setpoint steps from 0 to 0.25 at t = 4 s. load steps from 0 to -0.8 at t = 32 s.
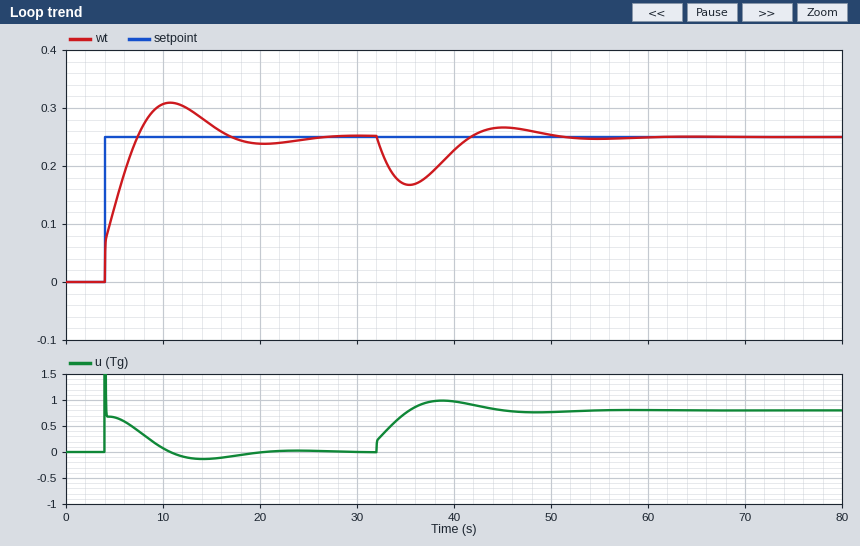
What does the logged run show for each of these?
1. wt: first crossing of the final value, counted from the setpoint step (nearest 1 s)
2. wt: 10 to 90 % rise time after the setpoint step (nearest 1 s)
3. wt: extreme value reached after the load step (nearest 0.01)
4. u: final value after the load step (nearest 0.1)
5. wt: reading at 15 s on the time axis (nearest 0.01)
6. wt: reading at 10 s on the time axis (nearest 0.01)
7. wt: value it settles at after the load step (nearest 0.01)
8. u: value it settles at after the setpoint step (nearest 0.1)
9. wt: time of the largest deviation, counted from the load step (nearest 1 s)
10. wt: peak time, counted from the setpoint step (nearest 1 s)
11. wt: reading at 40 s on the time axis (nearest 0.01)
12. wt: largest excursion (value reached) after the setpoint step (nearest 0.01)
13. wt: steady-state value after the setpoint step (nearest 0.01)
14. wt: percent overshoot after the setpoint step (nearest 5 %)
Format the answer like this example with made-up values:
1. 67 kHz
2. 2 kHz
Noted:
1. 3 s
2. 3 s
3. 0.17
4. 0.8
5. 0.27
6. 0.31
7. 0.25
8. 0.0
9. 3 s
10. 7 s
11. 0.23
12. 0.31
13. 0.25
14. 25 %
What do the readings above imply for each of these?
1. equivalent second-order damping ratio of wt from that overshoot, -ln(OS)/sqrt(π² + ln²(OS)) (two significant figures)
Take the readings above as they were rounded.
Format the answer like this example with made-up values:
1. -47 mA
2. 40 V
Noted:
1. 0.40
